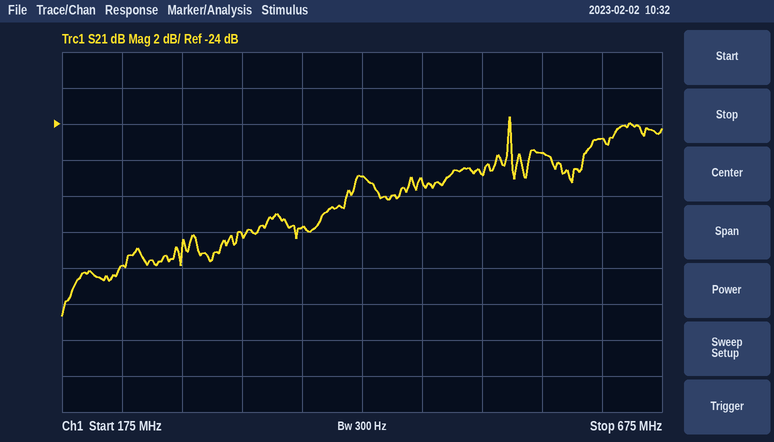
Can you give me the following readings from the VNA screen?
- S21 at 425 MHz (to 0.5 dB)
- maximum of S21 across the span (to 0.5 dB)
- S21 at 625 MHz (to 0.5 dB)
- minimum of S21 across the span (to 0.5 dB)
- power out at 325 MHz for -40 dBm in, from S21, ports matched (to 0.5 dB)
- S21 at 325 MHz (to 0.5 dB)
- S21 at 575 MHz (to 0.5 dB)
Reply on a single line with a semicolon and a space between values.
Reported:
-27.0 dB; -23.5 dB; -25.0 dB; -34.5 dB; -70.0 dBm; -30.0 dB; -25.5 dB
